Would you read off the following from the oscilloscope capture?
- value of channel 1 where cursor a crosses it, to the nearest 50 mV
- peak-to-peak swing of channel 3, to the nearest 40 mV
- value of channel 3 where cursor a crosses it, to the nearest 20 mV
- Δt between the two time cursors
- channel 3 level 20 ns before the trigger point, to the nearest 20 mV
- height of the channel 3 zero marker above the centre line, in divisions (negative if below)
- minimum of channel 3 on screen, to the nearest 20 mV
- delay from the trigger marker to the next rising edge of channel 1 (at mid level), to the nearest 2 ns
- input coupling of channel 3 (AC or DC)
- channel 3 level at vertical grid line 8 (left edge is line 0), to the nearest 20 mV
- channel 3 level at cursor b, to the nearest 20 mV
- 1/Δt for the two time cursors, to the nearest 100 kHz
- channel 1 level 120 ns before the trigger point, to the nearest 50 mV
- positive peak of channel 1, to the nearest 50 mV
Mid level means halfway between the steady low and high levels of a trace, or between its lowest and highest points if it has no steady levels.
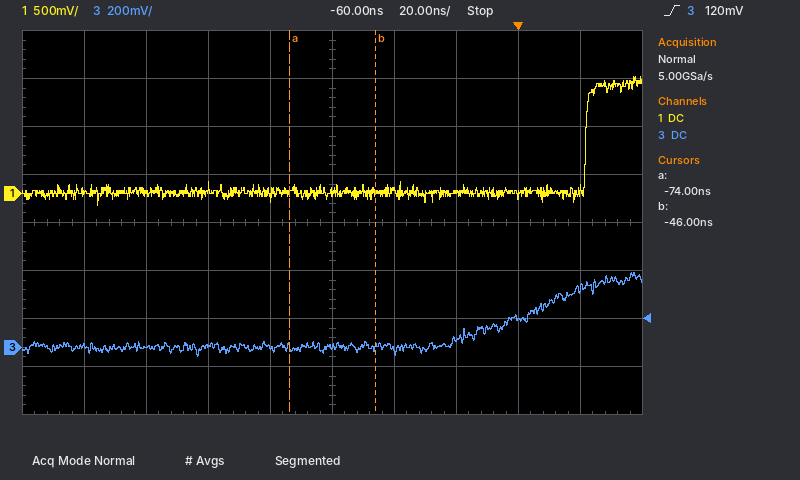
0 mV
360 mV
0 mV
28 ns
40 mV
-2.6 div
-40 mV
22 ns
DC
120 mV
0 mV
35.7 MHz
0 mV
1.20 V
